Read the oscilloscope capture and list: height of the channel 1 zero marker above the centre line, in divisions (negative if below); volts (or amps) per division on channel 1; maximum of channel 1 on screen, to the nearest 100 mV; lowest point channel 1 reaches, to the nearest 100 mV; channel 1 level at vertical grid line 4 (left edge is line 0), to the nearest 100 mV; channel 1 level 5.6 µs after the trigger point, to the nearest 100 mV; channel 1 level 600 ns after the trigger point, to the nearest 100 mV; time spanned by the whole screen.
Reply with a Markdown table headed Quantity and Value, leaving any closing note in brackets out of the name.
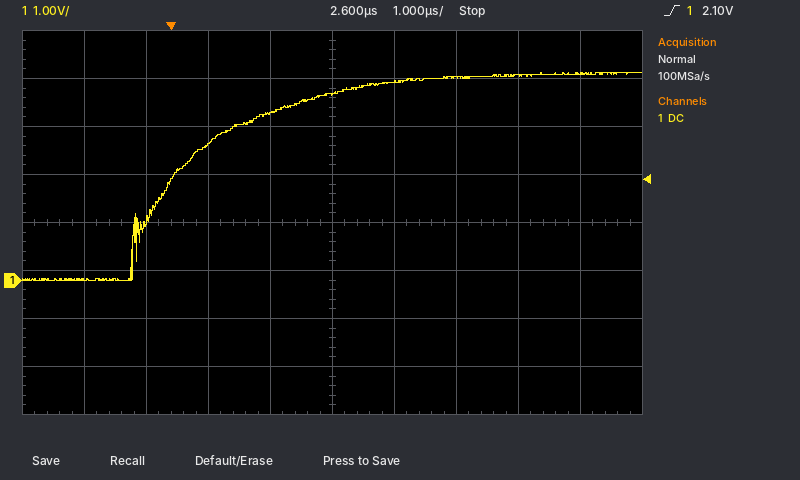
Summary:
| Quantity | Value |
|---|---|
| height of the channel 1 zero marker above the centre line, in divisions | -1.2 div |
| volts (or amps) per division on channel 1 | 1 V |
| maximum of channel 1 on screen, to the nearest 100 mV | 4.3 V |
| lowest point channel 1 reaches, to the nearest 100 mV | 0.0 V |
| channel 1 level at vertical grid line 4 (left edge is line 0), to the nearest 100 mV | 3.5 V |
| channel 1 level 5.6 µs after the trigger point, to the nearest 100 mV | 4.3 V |
| channel 1 level 600 ns after the trigger point, to the nearest 100 mV | 2.8 V |
| time spanned by the whole screen | 10 µs |
